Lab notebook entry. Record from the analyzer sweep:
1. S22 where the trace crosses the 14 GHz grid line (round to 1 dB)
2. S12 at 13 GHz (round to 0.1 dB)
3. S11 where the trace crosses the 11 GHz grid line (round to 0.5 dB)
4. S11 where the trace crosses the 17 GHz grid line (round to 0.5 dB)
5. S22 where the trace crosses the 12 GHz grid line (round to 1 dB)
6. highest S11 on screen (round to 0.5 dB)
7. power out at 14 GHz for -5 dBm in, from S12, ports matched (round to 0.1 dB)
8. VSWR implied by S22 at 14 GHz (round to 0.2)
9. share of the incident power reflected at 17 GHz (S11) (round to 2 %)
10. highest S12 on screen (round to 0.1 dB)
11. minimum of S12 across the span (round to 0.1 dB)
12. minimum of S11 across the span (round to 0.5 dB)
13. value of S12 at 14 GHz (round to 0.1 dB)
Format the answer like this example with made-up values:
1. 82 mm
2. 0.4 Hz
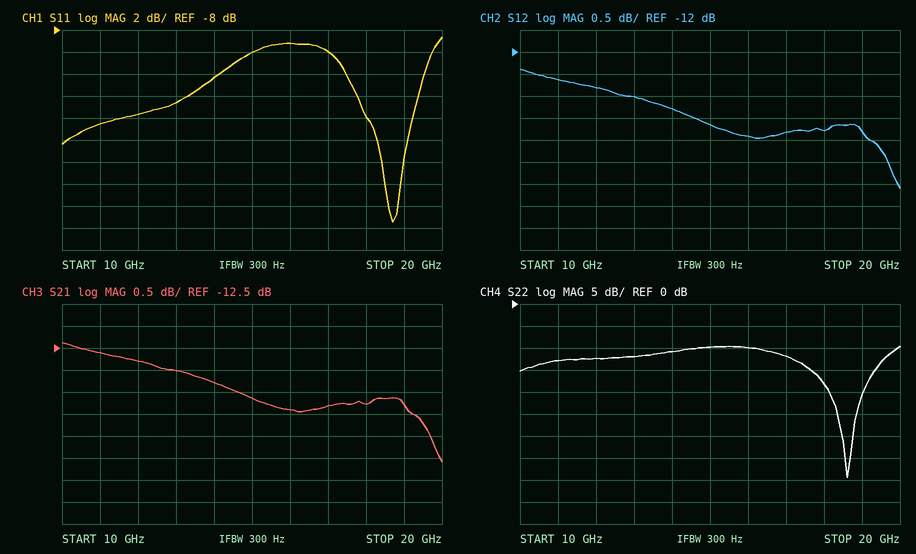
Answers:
1. -11 dB
2. -13.0 dB
3. -16.5 dB
4. -10.0 dB
5. -12 dB
6. -8.5 dB
7. -18.3 dBm
8. 1.8
9. 10 %
10. -12.4 dB
11. -15.1 dB
12. -25.5 dB
13. -13.3 dB
